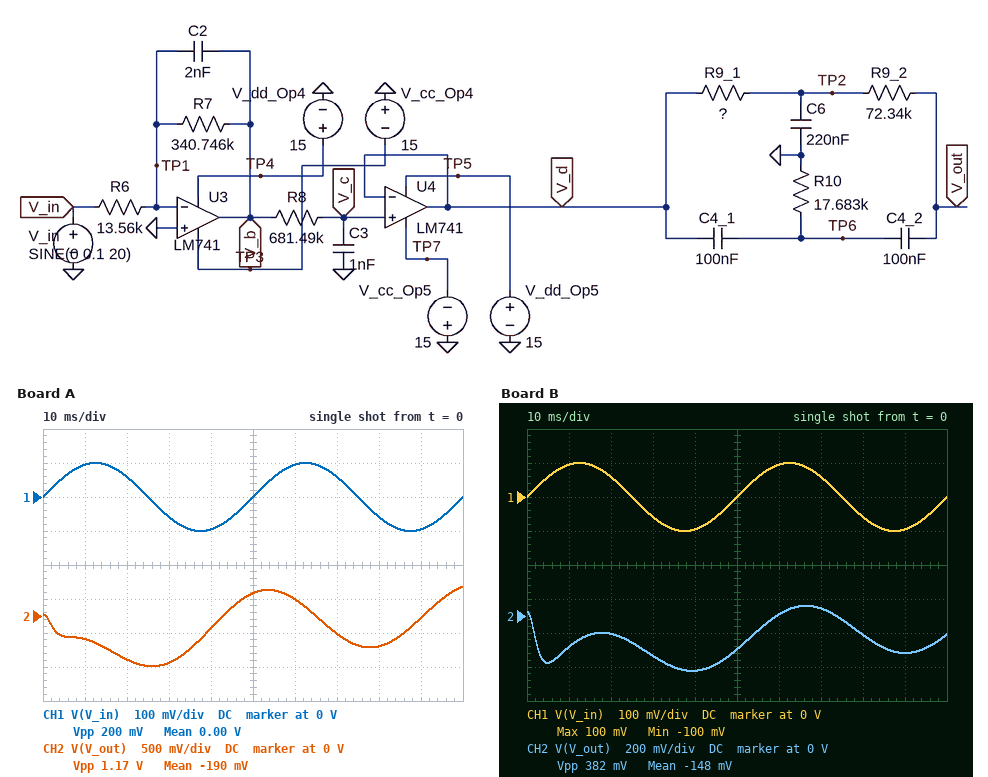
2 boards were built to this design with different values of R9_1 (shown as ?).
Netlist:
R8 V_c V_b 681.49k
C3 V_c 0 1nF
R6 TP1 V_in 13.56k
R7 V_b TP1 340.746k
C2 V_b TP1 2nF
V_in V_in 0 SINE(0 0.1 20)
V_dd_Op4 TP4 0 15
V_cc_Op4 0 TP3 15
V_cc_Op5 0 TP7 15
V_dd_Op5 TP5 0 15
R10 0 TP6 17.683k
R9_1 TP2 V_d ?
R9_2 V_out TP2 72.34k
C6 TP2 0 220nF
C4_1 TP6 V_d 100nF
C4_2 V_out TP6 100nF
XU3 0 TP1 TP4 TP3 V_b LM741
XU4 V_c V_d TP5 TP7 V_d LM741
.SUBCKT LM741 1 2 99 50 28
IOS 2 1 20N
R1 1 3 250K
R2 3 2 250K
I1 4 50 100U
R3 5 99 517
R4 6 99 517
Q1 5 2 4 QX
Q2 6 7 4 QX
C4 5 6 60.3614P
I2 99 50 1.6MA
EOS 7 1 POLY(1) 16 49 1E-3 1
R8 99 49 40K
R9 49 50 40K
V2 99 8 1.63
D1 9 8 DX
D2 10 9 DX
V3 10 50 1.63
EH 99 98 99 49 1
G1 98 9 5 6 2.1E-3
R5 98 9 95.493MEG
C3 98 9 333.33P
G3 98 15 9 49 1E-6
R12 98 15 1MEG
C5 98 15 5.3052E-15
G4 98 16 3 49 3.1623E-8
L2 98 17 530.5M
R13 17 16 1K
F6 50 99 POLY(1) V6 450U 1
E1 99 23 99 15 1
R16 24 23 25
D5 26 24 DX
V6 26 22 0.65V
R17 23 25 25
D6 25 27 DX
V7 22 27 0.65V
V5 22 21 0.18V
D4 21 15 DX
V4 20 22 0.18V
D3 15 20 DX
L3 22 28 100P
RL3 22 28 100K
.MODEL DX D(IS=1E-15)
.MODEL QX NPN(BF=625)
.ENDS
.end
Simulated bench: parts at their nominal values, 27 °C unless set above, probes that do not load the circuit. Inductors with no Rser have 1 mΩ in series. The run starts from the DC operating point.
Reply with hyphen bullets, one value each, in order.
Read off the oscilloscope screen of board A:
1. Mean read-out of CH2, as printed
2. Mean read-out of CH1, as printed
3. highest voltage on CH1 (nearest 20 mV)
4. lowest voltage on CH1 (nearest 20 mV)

- -190 mV
- 0.00 V
- 100 mV
- -100 mV
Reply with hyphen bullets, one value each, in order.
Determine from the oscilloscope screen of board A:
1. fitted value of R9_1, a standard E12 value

- 56 kΩ
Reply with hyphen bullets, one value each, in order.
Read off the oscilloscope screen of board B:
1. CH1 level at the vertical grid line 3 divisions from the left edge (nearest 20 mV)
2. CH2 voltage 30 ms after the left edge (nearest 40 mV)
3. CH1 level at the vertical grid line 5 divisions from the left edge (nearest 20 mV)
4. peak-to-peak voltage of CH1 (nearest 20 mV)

- -60 mV
- -240 mV
- 0 V
- 200 mV
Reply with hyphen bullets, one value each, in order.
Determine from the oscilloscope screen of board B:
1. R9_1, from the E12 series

- 180 kΩ
